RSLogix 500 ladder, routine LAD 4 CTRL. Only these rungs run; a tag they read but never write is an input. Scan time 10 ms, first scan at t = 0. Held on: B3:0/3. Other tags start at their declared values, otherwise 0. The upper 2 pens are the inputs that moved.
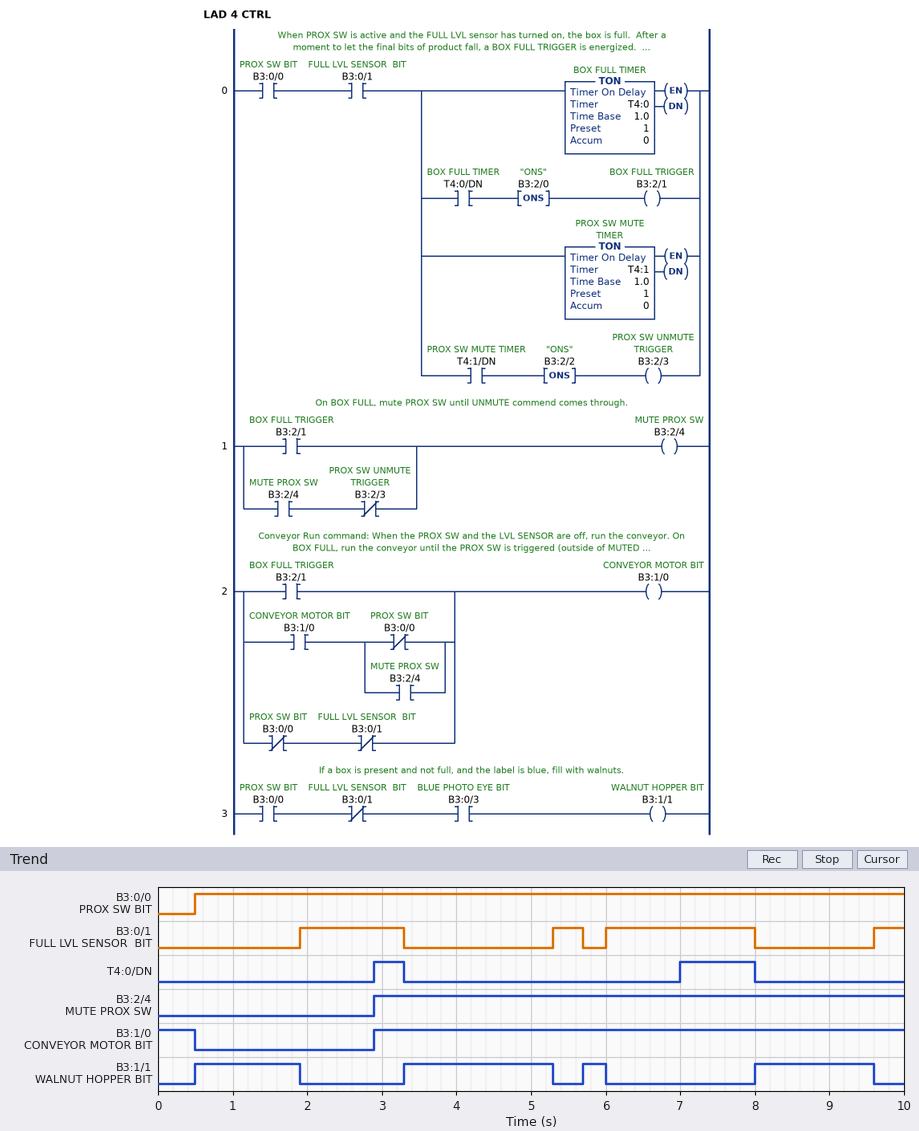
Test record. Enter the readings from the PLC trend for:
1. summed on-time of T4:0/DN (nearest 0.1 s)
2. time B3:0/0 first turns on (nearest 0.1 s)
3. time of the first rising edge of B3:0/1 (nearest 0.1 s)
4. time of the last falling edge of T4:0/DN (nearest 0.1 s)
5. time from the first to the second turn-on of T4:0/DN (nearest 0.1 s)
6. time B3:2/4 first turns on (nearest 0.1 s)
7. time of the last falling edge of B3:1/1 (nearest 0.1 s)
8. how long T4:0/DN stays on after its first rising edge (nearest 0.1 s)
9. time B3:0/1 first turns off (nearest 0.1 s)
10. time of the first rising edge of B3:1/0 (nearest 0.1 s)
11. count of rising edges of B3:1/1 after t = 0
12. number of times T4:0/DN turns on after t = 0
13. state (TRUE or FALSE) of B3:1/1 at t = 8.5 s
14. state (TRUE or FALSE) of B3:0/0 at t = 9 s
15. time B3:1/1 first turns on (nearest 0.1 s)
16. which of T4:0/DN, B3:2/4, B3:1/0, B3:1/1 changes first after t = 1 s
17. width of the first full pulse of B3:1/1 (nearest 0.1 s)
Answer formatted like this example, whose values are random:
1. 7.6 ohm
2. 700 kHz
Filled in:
1. 1.4 s
2. 0.5 s
3. 1.9 s
4. 8.0 s
5. 4.1 s
6. 2.9 s
7. 9.6 s
8. 0.4 s
9. 3.3 s
10. 2.9 s
11. 4
12. 2
13. TRUE
14. TRUE
15. 0.5 s
16. B3:1/1
17. 1.4 s
